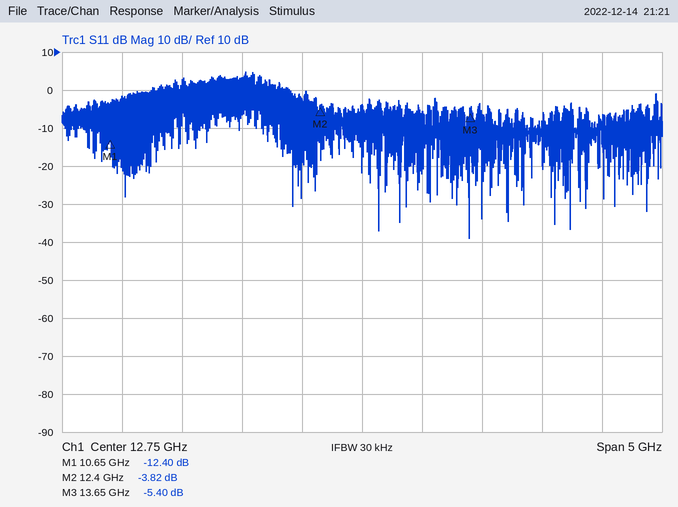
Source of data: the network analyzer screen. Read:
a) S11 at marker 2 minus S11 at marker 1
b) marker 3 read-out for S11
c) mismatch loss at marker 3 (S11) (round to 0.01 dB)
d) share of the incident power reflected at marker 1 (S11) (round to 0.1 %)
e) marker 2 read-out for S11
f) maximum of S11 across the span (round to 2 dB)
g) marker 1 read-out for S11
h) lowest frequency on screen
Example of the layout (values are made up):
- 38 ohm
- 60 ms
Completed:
- 8.58 dB
- -5.40 dB
- 1.48 dB
- 5.8 %
- -3.82 dB
- 4 dB
- -12.40 dB
- 10.25 GHz
